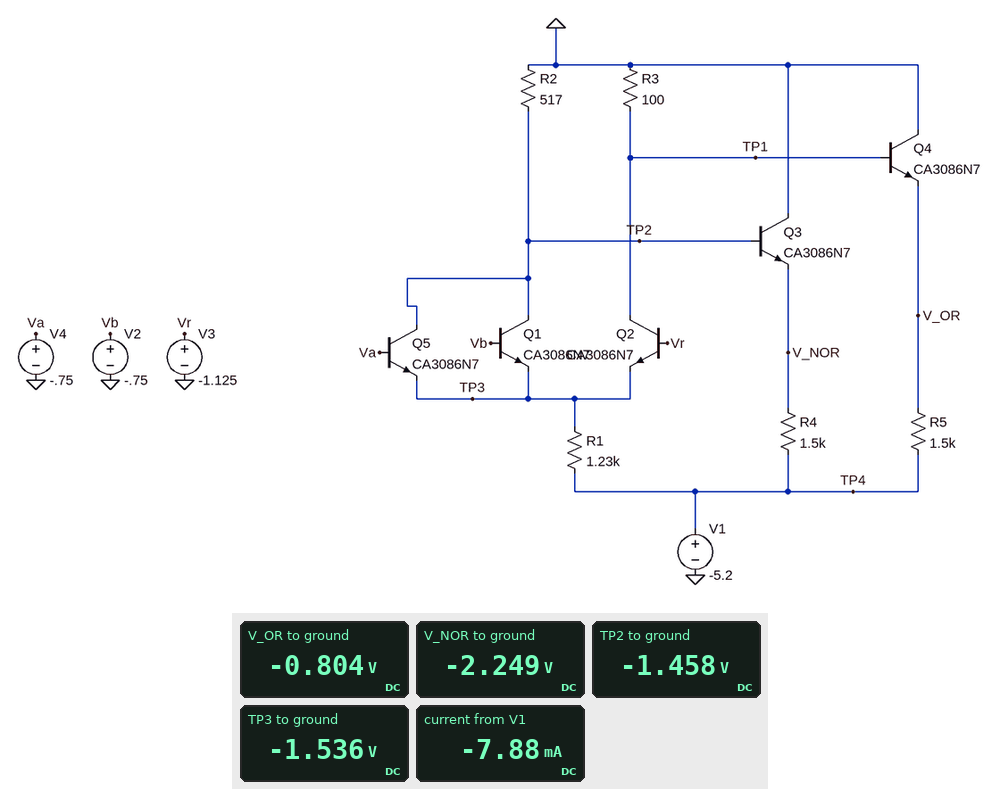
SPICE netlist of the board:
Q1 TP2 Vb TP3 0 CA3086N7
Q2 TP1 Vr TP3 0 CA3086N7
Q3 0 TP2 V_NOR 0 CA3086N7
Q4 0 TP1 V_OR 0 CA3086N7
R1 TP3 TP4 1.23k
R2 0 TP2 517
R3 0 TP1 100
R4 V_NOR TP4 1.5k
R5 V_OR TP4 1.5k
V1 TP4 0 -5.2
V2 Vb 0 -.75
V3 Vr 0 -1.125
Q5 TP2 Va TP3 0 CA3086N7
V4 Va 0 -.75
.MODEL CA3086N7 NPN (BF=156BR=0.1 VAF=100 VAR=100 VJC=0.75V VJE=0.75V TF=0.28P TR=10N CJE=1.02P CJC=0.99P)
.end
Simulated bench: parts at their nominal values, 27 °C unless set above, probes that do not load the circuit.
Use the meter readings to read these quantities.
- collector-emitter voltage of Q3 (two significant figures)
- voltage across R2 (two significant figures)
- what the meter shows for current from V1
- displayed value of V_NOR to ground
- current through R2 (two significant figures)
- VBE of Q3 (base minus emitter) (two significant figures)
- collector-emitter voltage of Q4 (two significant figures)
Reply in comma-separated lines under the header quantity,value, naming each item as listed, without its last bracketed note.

quantity,value
collector-emitter voltage of Q3,2.2 V
voltage across R2,1.5 V
what the meter shows for current from V1,-7.88 mA
displayed value of V_NOR to ground,-2.249 V
current through R2,2.8 mA
VBE of Q3 (base minus emitter),790 mV
collector-emitter voltage of Q4,800 mV
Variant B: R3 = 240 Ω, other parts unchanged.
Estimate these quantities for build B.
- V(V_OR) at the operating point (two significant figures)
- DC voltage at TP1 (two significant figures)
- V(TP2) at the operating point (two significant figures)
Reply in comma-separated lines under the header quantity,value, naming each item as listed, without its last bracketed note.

quantity,value
V(V_OR) at the operating point,-810 mV
DC voltage at TP1,-4.5 mV
V(TP2) at the operating point,-1.5 V
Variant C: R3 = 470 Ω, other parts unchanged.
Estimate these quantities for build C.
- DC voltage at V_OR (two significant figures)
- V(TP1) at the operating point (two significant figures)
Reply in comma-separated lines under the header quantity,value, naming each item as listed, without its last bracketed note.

quantity,value
DC voltage at V_OR,-810 mV
V(TP1) at the operating point,-8.8 mV
